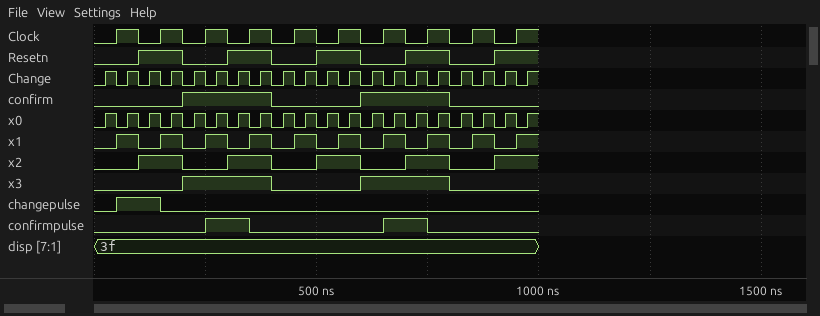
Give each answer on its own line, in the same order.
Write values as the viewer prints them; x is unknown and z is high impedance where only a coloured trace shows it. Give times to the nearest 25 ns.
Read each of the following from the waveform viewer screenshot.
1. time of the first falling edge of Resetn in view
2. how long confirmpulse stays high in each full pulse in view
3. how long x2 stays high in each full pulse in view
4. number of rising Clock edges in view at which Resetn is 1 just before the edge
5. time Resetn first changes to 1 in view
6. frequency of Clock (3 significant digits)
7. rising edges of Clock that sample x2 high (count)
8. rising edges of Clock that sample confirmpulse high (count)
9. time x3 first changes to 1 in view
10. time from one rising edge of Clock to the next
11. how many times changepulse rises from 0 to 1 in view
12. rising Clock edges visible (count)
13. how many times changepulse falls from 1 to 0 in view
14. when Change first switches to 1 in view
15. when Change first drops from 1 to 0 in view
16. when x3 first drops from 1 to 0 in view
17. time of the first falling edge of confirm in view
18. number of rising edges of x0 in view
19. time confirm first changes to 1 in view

200 ns
100 ns, 100 ns
100 ns, 100 ns, 100 ns, 100 ns
5
100 ns
10.0 MHz
5
2
200 ns
100 ns
1
10
1
25 ns
50 ns
400 ns
400 ns
20
200 ns
